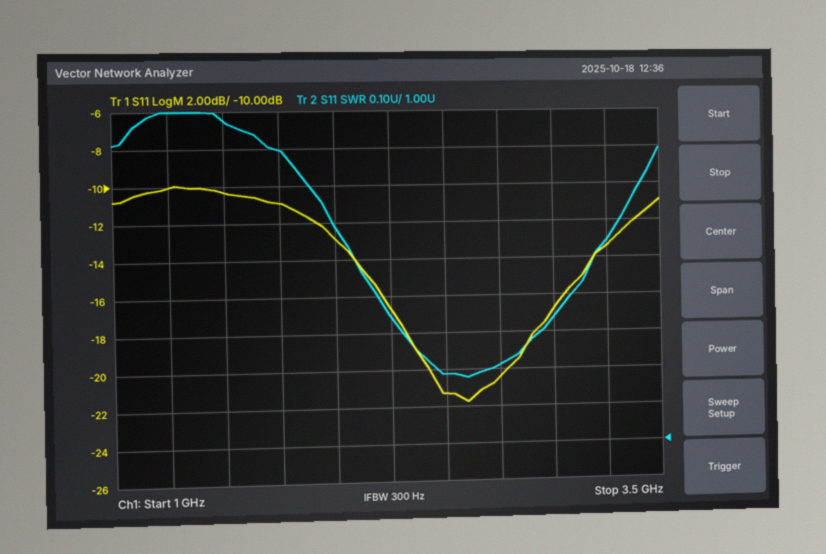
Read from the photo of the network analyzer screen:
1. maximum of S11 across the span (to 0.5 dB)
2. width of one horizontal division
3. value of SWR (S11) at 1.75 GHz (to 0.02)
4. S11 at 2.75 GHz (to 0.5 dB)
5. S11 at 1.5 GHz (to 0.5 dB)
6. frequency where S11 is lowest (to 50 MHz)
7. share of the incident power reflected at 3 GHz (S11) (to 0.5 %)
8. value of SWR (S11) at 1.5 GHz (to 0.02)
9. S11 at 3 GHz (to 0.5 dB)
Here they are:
-10.0 dB
250 MHz
1.80
-20.5 dB
-10.5 dB
2.60 GHz
2.0 %
1.88
-17.0 dB
